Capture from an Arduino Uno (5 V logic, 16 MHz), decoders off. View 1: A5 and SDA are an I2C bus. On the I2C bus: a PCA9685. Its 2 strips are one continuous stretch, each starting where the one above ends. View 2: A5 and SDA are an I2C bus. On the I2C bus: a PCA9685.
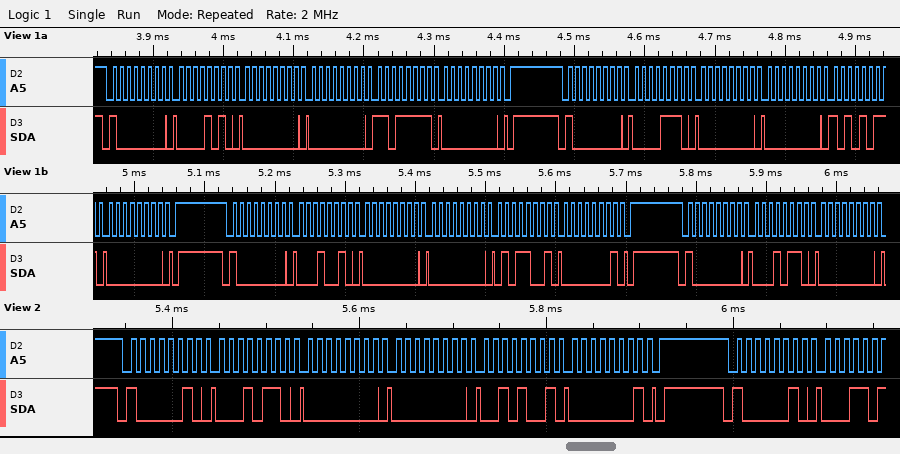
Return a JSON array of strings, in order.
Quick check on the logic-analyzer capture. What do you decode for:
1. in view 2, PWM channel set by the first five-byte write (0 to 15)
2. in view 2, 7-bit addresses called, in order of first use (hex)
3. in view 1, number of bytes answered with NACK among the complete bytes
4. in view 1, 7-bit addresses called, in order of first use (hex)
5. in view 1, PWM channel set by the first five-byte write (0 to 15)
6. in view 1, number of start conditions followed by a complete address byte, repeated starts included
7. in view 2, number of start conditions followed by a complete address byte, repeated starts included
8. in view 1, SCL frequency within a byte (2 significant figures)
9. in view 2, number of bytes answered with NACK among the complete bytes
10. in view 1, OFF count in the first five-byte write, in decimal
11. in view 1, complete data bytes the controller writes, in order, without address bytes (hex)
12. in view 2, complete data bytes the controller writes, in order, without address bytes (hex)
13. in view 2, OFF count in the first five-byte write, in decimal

["4", "0x41", "0", "0x40", "1", "4", "2", "100 kHz", "0", "223", "0A 00 00 DF 00 0E 00 00 AB 00 12 00 00 59 01 16 00", "16 00 00 29 01", "297"]
